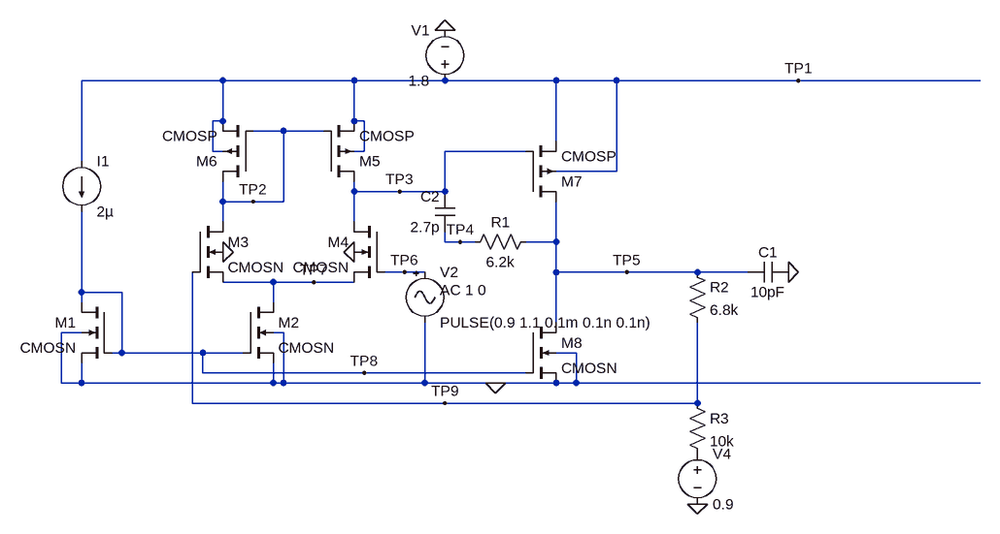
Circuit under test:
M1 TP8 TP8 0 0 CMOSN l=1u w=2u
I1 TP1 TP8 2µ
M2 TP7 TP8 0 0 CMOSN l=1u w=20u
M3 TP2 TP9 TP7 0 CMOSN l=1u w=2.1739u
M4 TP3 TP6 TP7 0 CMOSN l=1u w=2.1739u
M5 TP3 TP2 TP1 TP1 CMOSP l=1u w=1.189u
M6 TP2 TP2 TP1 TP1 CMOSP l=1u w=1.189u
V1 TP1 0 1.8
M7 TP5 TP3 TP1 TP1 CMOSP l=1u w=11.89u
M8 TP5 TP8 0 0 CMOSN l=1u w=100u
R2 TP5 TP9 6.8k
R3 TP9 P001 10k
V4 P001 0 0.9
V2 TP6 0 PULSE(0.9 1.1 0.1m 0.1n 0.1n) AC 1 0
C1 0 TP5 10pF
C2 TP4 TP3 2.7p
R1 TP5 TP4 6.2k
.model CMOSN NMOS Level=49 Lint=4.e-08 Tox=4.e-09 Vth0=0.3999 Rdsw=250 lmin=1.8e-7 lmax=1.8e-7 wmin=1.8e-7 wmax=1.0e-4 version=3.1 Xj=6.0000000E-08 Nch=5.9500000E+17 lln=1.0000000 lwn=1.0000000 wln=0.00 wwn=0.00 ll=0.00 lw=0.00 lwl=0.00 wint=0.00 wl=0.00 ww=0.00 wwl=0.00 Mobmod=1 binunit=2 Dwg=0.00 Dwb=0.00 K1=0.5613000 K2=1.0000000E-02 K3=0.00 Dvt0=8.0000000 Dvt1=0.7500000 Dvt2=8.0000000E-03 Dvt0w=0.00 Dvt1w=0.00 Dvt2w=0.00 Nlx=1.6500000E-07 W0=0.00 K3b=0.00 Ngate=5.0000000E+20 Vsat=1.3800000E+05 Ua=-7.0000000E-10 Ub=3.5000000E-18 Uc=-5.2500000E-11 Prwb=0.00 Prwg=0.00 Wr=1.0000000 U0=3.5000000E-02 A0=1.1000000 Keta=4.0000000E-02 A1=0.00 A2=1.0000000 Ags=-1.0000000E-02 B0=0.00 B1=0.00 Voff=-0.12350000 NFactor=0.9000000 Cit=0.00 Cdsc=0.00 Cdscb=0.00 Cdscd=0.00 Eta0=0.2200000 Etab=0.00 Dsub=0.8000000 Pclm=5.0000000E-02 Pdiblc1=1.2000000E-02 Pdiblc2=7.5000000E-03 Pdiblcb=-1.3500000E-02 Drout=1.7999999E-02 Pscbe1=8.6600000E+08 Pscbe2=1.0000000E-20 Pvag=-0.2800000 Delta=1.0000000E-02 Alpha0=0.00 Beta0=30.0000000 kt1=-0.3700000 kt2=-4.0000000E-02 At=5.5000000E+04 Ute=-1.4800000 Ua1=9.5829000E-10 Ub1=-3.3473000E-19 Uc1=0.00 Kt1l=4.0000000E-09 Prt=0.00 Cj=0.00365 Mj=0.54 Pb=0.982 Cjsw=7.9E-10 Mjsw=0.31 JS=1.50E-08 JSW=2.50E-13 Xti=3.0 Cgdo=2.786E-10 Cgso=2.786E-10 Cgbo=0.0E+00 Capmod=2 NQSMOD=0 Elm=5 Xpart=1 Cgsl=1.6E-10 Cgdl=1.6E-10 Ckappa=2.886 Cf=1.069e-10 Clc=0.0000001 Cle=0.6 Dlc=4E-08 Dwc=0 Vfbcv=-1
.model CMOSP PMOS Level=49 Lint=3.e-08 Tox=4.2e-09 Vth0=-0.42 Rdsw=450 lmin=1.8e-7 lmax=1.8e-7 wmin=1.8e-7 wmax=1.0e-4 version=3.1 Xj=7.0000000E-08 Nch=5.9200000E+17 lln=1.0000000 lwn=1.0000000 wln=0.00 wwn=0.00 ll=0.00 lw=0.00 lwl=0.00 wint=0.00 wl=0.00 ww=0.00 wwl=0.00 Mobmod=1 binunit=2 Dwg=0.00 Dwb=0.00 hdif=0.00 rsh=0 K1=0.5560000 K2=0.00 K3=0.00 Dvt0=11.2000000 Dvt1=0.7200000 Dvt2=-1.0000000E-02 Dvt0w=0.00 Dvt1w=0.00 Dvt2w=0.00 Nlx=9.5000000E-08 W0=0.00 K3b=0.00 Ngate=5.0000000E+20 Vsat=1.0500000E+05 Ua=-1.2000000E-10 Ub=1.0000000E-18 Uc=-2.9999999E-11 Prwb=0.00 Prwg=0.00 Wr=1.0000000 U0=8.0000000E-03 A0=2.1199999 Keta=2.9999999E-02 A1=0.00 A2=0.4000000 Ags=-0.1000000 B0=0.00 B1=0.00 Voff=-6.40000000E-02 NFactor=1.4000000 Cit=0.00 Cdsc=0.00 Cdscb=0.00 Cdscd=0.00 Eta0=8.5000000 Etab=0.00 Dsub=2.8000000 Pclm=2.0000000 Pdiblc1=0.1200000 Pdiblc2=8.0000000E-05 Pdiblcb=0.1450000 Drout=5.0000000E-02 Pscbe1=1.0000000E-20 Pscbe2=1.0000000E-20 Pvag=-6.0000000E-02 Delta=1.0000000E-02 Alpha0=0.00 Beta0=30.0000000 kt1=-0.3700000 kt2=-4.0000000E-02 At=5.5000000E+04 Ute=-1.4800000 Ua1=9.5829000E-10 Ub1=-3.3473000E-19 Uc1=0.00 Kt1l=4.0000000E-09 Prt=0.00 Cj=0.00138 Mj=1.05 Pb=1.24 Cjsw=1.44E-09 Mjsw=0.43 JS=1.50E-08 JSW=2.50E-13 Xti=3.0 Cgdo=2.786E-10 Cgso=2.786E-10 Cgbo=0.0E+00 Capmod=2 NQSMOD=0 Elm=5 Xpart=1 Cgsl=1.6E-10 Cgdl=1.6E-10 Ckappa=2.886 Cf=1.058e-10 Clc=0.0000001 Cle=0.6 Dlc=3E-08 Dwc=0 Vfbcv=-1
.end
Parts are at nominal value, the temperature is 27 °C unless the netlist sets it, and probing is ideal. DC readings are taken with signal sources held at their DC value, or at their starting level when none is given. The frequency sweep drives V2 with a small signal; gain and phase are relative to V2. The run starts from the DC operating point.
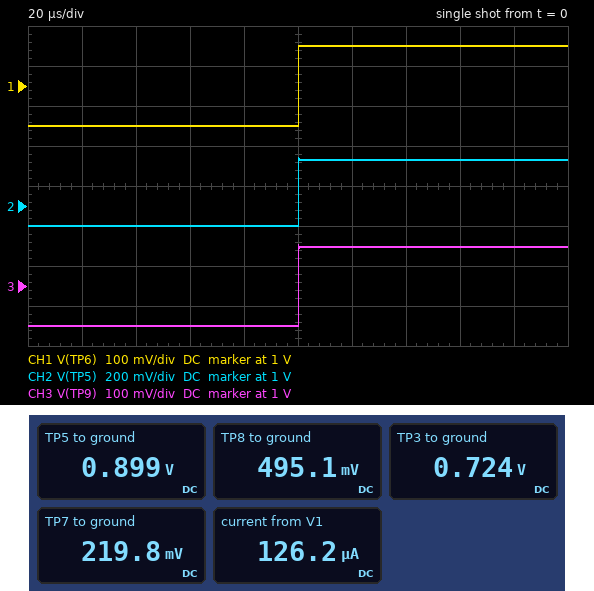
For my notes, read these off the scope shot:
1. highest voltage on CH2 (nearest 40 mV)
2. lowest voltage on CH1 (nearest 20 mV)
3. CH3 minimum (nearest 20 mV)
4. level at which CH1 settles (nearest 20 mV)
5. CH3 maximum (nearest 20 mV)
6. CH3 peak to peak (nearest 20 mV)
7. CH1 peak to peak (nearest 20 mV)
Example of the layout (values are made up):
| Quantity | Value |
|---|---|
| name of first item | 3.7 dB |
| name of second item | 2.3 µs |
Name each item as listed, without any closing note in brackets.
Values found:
| Quantity | Value |
|---|---|
| highest voltage on CH2 | 1.24 V |
| lowest voltage on CH1 | 900 mV |
| CH3 minimum | 900 mV |
| level at which CH1 settles | 1.10 V |
| CH3 maximum | 1.10 V |
| CH3 peak to peak | 200 mV |
| CH1 peak to peak | 200 mV |
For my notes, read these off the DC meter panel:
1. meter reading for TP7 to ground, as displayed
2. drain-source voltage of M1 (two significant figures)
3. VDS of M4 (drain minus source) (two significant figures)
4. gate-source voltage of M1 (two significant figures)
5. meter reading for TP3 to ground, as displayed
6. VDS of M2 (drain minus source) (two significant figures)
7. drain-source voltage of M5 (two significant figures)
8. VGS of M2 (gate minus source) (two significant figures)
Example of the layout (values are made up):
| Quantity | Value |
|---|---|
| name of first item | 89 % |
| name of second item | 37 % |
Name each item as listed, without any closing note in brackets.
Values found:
| Quantity | Value |
|---|---|
| meter reading for TP7 to ground, as displayed | 219.8 mV |
| drain-source voltage of M1 | 500 mV |
| VDS of M4 (drain minus source) | 500 mV |
| gate-source voltage of M1 | 500 mV |
| meter reading for TP3 to ground, as displayed | 0.724 V |
| VDS of M2 (drain minus source) | 220 mV |
| drain-source voltage of M5 | -1.1 V |
| VGS of M2 (gate minus source) | 500 mV |
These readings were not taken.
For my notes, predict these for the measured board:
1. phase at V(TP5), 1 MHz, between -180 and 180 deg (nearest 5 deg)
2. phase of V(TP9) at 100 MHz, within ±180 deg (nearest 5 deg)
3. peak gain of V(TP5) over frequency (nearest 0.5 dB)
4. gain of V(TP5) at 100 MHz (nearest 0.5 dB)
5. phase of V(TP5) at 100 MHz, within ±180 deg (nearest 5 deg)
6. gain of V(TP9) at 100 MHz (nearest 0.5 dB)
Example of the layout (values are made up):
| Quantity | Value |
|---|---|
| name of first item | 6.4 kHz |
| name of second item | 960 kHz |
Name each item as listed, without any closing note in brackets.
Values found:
| Quantity | Value |
|---|---|
| phase at V(TP5), 1 MHz, between -180 and 180 deg | -25 deg |
| phase of V(TP9) at 100 MHz, within ±180 deg | 90 deg |
| peak gain of V(TP5) over frequency | 4.5 dB |
| gain of V(TP5) at 100 MHz | -41.5 dB |
| phase of V(TP5) at 100 MHz, within ±180 deg | -135 deg |
| gain of V(TP9) at 100 MHz | -37.5 dB |
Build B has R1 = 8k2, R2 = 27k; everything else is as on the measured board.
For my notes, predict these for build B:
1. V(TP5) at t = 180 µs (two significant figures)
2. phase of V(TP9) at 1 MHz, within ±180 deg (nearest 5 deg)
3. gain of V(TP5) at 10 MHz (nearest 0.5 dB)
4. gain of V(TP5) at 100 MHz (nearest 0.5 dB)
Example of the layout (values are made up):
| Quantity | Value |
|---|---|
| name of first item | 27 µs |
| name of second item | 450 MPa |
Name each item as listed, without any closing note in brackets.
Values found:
| Quantity | Value |
|---|---|
| V(TP5) at t = 180 µs | 1.5 V |
| phase of V(TP9) at 1 MHz, within ±180 deg | -45 deg |
| gain of V(TP5) at 10 MHz | -12.5 dB |
| gain of V(TP5) at 100 MHz | -37.0 dB |
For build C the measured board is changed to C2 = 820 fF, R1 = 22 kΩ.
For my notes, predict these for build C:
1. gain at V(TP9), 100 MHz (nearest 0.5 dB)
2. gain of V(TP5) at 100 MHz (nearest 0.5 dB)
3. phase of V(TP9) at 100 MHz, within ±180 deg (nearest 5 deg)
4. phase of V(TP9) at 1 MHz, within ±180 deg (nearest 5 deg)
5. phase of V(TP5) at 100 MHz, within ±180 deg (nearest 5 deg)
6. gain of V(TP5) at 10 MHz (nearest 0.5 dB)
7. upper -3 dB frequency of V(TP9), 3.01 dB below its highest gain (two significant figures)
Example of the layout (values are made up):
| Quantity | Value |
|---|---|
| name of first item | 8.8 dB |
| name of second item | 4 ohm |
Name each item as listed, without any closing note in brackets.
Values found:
| Quantity | Value |
|---|---|
| gain at V(TP9), 100 MHz | -34.0 dB |
| gain of V(TP5) at 100 MHz | -28.0 dB |
| phase of V(TP9) at 100 MHz, within ±180 deg | 160 deg |
| phase of V(TP9) at 1 MHz, within ±180 deg | -10 deg |
| phase of V(TP5) at 100 MHz, within ±180 deg | -155 deg |
| gain of V(TP5) at 10 MHz | -2.0 dB |
| upper -3 dB frequency of V(TP9), 3.01 dB below its highest gain | 6.7 MHz |
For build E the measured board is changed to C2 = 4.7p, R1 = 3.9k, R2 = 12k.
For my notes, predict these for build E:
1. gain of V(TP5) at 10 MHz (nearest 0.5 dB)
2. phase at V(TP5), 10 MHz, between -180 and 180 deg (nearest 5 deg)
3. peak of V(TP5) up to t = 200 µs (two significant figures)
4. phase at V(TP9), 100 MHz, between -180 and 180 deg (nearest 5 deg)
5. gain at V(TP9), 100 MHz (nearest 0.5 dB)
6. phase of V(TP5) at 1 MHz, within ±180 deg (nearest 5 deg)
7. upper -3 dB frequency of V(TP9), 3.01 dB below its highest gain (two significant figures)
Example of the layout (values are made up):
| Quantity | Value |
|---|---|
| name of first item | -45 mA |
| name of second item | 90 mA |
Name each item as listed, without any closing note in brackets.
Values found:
| Quantity | Value |
|---|---|
| gain of V(TP5) at 10 MHz | -19.0 dB |
| phase at V(TP5), 10 MHz, between -180 and 180 deg | -145 deg |
| peak of V(TP5) up to t = 200 µs | 1.3 V |
| phase at V(TP9), 100 MHz, between -180 and 180 deg | 80 deg |
| gain at V(TP9), 100 MHz | -33.0 dB |
| phase of V(TP5) at 1 MHz, within ±180 deg | -50 deg |
| upper -3 dB frequency of V(TP9), 3.01 dB below its highest gain | 1.3 MHz |
